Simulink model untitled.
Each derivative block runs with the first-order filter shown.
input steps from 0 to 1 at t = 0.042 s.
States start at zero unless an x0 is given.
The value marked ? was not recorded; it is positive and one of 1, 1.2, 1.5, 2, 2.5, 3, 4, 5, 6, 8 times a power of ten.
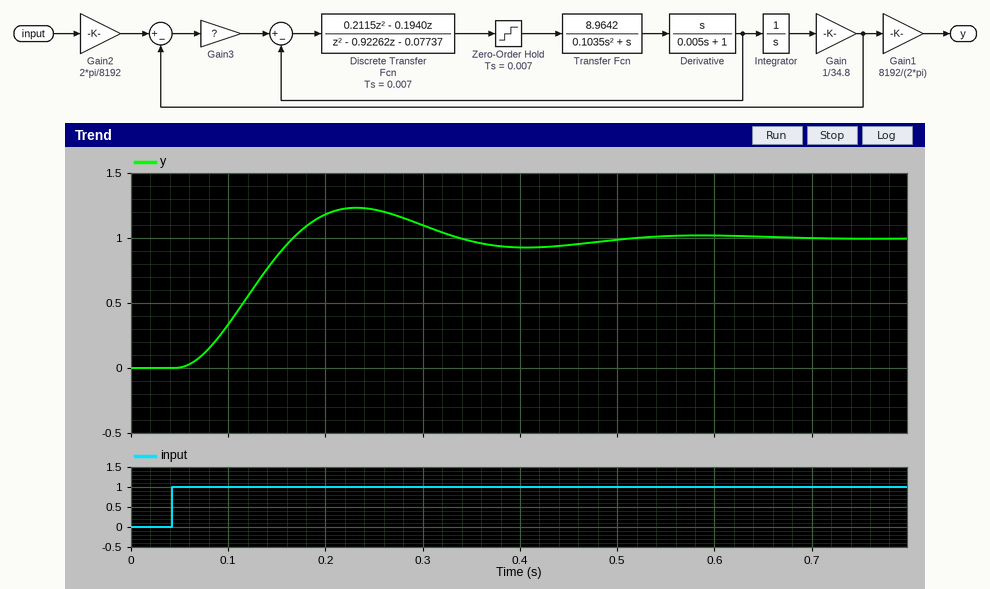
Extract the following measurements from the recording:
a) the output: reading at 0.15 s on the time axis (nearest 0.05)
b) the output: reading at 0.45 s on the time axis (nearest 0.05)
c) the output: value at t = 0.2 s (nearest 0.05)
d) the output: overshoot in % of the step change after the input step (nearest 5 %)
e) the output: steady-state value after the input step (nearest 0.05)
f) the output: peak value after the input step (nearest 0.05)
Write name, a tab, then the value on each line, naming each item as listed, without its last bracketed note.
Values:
the output: reading at 0.15 s on the time axis	0.85
the output: reading at 0.45 s on the time axis	0.95
the output: value at t = 0.2 s	1.20
the output: overshoot in % of the step change after the input step	25 %
the output: steady-state value after the input step	1.00
the output: peak value after the input step	1.25
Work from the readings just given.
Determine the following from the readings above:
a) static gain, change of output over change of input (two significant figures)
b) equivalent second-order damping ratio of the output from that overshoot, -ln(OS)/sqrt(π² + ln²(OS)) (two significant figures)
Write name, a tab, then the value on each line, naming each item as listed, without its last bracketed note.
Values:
static gain, change of output over change of input	1.0
equivalent second-order damping ratio of the output from that overshoot, -ln(OS)/sqrt(π² + ln²(OS))	0.40
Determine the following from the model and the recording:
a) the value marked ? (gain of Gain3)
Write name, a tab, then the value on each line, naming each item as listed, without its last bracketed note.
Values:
the value marked ?	600
